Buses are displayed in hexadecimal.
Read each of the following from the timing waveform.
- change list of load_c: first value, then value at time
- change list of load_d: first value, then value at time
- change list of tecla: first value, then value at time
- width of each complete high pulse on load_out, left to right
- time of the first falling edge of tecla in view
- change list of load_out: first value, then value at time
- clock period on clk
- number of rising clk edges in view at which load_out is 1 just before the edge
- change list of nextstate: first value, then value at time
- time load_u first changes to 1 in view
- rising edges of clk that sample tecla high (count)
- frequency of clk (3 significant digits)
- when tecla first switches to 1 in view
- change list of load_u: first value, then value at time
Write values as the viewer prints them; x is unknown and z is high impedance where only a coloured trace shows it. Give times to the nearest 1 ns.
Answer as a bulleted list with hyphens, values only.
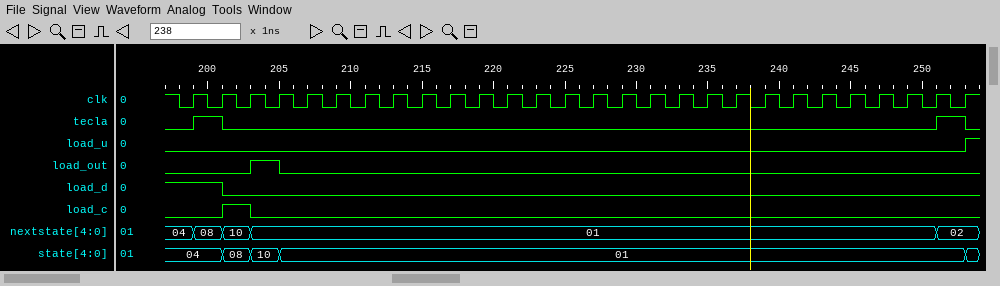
- 0, 1 at 201 ns, 0 at 203 ns
- 1, 0 at 201 ns
- 0, 1 at 199 ns, 0 at 201 ns, 1 at 251 ns, 0 at 253 ns
- 2 ns
- 201 ns
- 0, 1 at 203 ns, 0 at 205 ns
- 2 ns
- 1
- 04, 08 at 199 ns, 10 at 201 ns, 01 at 203 ns, 02 at 251 ns
- 253 ns
- 2
- 500 MHz
- 199 ns
- 0, 1 at 253 ns
